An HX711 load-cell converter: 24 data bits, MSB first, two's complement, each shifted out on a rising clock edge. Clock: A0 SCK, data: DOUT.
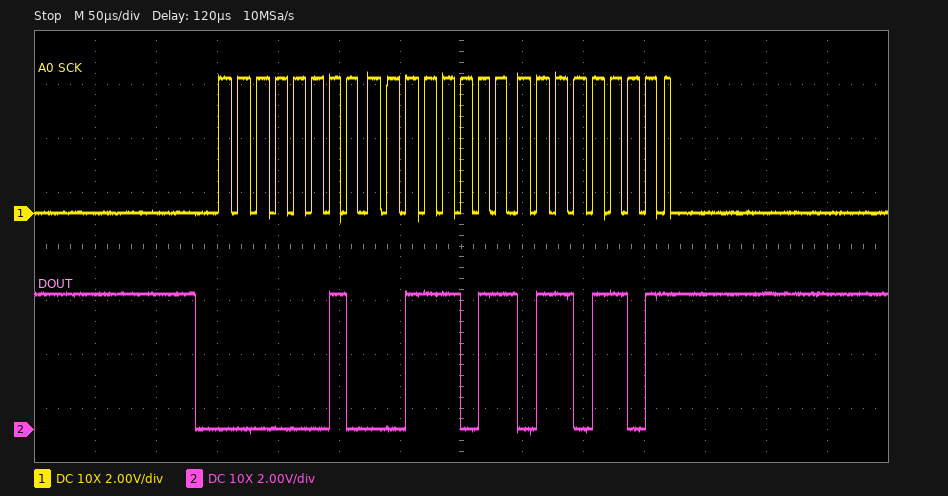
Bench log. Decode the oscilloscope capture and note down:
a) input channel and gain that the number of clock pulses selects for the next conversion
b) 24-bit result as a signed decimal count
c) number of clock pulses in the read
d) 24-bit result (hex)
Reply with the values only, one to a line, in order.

channel A, gain 128
146285
25
0x023B6D
